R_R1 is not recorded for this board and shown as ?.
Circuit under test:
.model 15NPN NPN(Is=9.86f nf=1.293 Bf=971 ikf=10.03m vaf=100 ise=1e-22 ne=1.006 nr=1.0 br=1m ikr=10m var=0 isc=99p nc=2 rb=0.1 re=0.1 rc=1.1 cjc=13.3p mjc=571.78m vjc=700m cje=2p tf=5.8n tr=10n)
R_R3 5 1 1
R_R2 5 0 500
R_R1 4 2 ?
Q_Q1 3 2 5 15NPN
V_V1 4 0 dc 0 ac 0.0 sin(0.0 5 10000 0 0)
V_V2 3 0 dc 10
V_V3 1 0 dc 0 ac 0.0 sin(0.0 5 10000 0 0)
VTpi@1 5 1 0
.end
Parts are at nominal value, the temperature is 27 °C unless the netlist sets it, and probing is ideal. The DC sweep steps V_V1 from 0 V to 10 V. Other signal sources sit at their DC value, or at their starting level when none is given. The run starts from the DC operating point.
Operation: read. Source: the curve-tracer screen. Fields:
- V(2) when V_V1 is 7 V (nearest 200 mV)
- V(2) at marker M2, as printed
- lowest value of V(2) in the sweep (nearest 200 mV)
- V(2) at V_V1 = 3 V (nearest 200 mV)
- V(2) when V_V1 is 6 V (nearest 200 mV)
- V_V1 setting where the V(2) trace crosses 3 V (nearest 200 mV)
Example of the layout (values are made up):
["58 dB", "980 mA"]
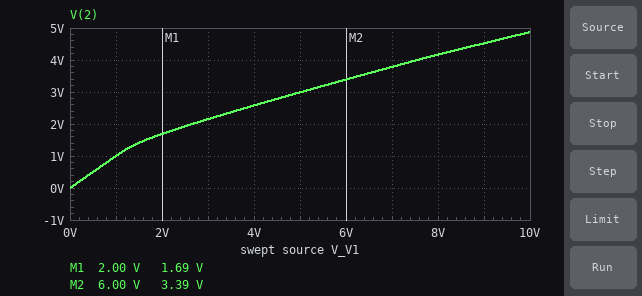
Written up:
["3.8 V", "3.39 V", "0 V", "2.2 V", "3.4 V", "5.0 V"]
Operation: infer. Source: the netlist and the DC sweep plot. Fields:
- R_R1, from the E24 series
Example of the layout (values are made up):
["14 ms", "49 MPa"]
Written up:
["0.36 Ω"]
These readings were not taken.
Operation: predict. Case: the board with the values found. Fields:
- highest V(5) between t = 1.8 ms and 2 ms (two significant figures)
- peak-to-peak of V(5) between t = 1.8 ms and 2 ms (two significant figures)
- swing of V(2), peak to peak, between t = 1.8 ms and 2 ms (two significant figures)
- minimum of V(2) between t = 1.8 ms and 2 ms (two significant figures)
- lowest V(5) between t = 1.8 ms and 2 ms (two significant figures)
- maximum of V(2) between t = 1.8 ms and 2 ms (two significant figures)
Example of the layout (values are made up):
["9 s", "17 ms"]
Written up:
["5.0 V", "10 V", "10 V", "-5.0 V", "-5.0 V", "5.0 V"]
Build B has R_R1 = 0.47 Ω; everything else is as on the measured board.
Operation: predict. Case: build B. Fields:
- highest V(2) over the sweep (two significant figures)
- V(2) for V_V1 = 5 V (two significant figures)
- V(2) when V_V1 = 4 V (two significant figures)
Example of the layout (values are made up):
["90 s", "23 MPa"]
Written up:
["4.4 V", "2.8 V", "2.4 V"]
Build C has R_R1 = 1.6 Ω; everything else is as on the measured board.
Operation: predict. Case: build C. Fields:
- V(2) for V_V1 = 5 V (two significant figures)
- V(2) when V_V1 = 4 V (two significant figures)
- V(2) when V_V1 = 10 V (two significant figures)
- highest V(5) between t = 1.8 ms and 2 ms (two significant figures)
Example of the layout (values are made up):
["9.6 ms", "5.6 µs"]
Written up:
["2.0 V", "1.9 V", "2.7 V", "5.0 V"]
